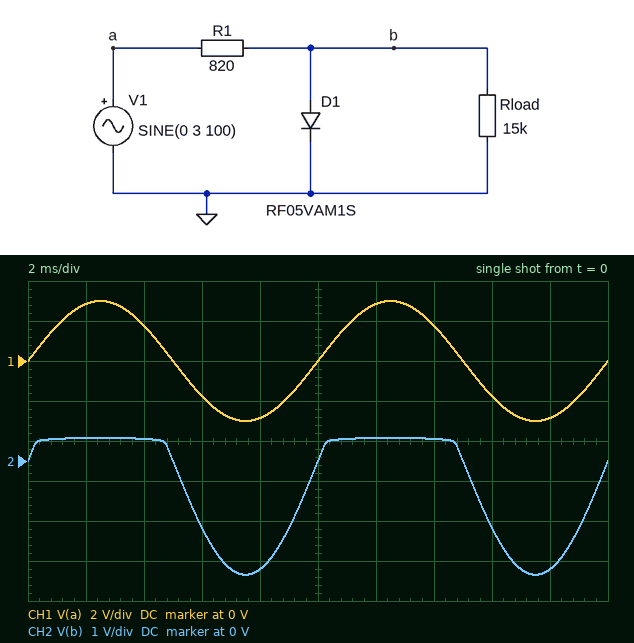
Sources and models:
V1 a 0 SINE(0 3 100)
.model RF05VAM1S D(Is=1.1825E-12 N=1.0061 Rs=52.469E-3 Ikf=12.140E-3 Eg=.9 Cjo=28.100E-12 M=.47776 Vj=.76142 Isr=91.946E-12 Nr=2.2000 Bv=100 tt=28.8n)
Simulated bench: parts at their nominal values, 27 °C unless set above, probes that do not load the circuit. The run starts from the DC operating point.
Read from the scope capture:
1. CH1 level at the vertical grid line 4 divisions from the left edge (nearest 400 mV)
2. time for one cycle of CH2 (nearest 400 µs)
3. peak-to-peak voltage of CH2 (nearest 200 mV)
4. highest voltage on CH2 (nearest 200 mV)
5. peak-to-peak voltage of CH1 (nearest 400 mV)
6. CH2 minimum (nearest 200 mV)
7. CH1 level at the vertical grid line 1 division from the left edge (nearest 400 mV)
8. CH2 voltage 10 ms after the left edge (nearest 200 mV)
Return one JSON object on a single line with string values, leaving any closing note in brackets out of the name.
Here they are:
{"CH1 level at the vertical grid line 4 divisions from the left edge": "-2.8 V", "time for one cycle of CH2": "10.0 ms", "peak-to-peak voltage of CH2": "3.4 V", "highest voltage on CH2": "600 mV", "peak-to-peak voltage of CH1": "6.0 V", "CH2 minimum": "-2.8 V", "CH1 level at the vertical grid line 1 division from the left edge": "2.8 V", "CH2 voltage 10 ms after the left edge": "0 V"}
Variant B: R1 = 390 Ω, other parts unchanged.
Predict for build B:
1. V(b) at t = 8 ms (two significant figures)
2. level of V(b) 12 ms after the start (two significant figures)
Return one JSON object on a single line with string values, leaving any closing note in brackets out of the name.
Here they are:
{"V(b) at t = 8 ms": "-2.8 V", "level of V(b) 12 ms after the start": "600 mV"}
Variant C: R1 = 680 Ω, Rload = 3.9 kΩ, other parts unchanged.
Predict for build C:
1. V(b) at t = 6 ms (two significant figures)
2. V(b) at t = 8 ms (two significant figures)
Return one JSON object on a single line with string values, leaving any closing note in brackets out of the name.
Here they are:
{"V(b) at t = 6 ms": "-1.5 V", "V(b) at t = 8 ms": "-2.4 V"}
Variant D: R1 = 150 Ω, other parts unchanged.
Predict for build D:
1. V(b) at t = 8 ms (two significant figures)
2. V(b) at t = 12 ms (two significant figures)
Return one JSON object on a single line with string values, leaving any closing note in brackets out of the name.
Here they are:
{"V(b) at t = 8 ms": "-2.8 V", "V(b) at t = 12 ms": "630 mV"}
